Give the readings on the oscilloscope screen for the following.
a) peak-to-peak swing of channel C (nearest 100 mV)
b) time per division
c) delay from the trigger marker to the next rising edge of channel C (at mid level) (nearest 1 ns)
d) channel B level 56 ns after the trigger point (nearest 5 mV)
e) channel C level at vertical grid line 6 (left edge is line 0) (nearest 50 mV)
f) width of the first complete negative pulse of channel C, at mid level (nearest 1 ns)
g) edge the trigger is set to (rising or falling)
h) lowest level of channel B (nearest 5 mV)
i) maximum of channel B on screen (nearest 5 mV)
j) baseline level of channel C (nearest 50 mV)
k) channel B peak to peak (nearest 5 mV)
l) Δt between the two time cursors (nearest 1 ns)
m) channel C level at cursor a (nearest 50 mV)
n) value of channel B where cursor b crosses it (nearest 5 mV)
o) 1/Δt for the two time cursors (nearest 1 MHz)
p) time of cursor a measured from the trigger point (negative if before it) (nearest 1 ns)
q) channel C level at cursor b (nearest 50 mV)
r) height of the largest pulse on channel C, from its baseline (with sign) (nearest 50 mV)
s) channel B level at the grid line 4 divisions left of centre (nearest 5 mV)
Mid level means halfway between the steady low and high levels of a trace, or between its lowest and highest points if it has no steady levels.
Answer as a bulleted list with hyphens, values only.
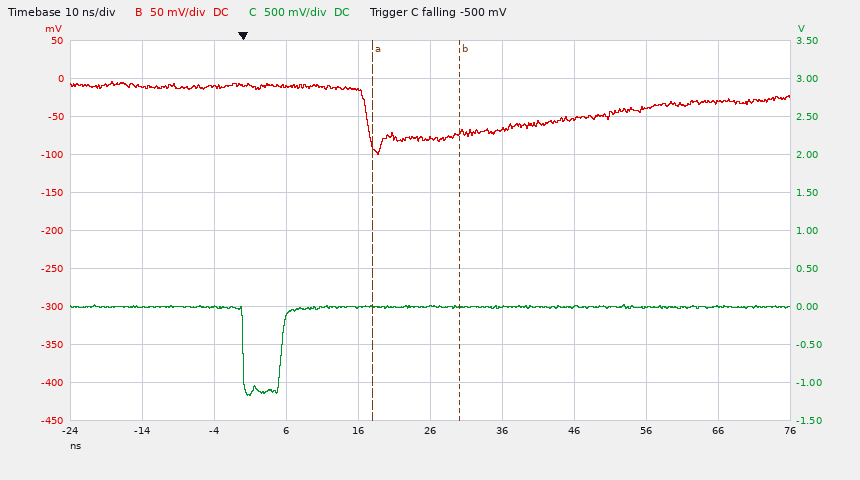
- 1.20 V
- 10 ns
- 5 ns
- -40 mV
- 0 mV
- 5 ns
- falling
- -100 mV
- -5 mV
- 0 mV
- 95 mV
- 12 ns
- 0 mV
- -70 mV
- 83 MHz
- +18 ns
- 0 mV
- -1.15 V
- -10 mV
